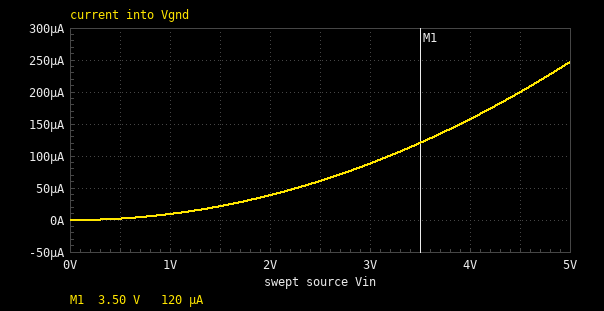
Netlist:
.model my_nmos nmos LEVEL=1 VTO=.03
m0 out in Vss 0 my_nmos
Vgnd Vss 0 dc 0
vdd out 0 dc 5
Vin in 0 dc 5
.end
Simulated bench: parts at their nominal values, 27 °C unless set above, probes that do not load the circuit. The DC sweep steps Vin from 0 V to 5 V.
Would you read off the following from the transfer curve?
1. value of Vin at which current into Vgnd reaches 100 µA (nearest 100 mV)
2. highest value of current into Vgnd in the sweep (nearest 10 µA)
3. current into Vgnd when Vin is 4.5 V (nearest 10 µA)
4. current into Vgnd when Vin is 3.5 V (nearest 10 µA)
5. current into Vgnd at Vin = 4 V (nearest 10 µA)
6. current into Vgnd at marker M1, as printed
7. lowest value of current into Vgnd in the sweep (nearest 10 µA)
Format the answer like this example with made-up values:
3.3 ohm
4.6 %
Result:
3.2 V
250 µA
200 µA
120 µA
160 µA
120 µA
0 A
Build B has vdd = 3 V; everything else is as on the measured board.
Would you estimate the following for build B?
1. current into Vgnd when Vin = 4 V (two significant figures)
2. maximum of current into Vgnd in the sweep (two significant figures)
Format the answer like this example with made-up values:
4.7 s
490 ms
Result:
150 µA
210 µA
